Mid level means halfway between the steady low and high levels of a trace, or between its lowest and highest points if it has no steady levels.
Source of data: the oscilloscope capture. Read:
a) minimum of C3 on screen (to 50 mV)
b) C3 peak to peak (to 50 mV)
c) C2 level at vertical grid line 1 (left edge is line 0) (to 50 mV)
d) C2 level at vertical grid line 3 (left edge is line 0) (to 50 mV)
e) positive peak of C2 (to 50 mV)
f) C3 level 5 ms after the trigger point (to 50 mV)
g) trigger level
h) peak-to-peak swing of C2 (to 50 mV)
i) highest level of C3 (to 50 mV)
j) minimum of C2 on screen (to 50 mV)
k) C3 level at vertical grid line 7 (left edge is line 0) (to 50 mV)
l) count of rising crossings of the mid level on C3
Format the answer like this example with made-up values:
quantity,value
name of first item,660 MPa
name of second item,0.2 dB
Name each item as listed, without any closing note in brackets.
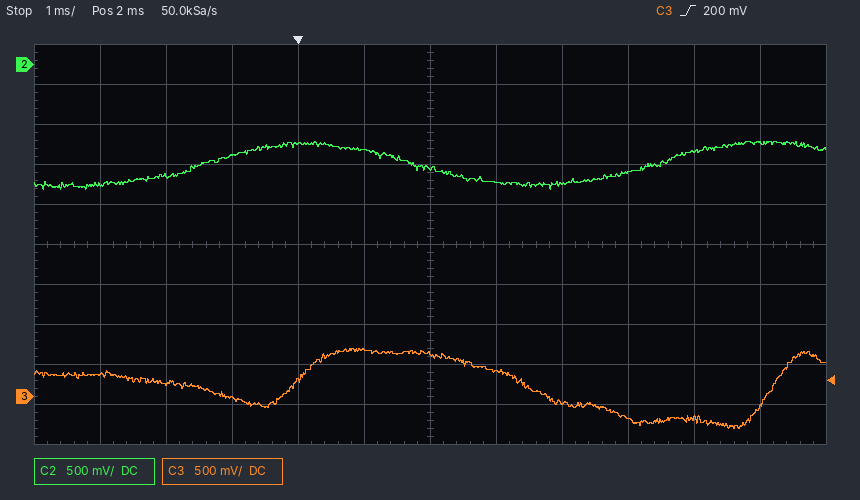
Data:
quantity,value
minimum of C3 on screen,-400 mV
C3 peak to peak,1.00 V
C2 level at vertical grid line 1 (left edge is line 0),-1.50 V
C2 level at vertical grid line 3 (left edge is line 0),-1.15 V
positive peak of C2,-950 mV
C3 level 5 ms after the trigger point,-250 mV
trigger level,200 mV
peak-to-peak swing of C2,600 mV
highest level of C3,600 mV
minimum of C2 on screen,-1.55 V
C3 level at vertical grid line 7 (left edge is line 0),300 mV
count of rising crossings of the mid level on C3,2
